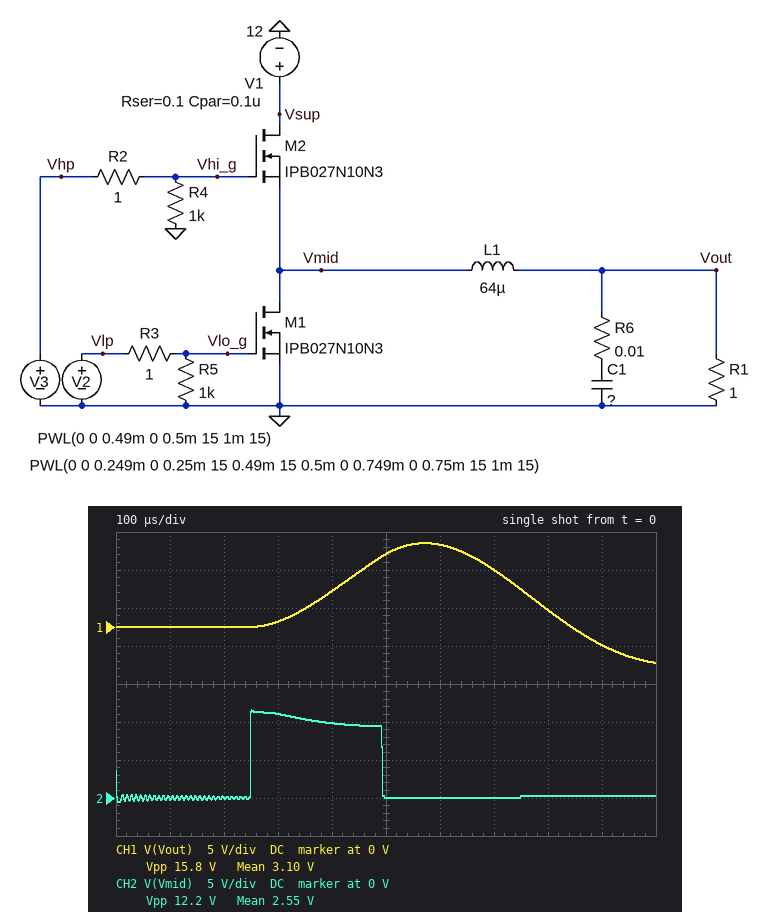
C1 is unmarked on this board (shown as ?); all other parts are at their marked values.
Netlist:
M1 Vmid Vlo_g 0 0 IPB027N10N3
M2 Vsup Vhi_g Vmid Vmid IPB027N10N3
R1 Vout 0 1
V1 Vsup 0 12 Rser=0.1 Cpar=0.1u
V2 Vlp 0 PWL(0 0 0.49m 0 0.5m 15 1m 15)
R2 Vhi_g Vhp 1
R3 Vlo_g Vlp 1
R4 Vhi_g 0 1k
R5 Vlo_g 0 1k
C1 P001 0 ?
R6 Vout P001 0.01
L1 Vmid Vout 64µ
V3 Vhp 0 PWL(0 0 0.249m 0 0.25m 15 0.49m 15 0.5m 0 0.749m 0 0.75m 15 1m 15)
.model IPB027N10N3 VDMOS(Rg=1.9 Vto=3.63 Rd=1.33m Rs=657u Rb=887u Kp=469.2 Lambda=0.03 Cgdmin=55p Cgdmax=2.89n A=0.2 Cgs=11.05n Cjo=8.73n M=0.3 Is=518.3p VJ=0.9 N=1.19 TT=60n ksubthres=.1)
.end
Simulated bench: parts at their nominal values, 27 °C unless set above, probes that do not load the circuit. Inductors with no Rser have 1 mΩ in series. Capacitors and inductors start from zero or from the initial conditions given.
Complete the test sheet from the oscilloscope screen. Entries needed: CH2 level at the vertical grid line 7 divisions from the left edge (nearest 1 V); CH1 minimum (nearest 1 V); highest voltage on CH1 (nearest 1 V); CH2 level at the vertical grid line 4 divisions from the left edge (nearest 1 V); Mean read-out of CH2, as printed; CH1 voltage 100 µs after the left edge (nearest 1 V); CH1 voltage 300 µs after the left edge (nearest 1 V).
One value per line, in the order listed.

0 V
-5 V
11 V
10 V
2.55 V
0 V
1 V
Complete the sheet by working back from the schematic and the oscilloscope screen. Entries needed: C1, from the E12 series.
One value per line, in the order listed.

330 µF
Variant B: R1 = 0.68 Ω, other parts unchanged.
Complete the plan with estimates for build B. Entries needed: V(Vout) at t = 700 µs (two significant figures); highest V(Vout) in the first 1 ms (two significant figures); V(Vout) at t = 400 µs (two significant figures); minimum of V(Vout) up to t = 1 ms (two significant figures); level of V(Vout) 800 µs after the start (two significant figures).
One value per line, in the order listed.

6.6 V
9.8 V
4.4 V
-2.8 V
2.4 V
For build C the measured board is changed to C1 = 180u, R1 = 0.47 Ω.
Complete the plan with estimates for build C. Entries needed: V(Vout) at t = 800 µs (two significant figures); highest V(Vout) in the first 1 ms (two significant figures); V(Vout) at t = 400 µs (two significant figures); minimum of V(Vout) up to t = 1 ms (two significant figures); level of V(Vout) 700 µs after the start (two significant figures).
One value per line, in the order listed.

590 mV
9.1 V
5.5 V
-500 mV
3.3 V
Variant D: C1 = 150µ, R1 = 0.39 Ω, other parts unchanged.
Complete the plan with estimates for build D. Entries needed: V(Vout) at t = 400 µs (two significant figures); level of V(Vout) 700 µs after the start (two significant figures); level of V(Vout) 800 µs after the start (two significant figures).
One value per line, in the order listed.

5.4 V
3.0 V
1.1 V
